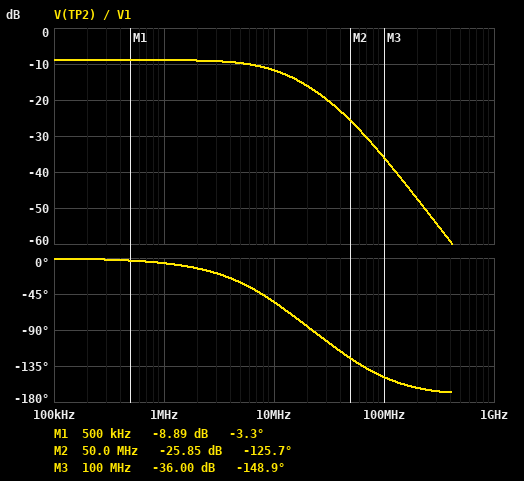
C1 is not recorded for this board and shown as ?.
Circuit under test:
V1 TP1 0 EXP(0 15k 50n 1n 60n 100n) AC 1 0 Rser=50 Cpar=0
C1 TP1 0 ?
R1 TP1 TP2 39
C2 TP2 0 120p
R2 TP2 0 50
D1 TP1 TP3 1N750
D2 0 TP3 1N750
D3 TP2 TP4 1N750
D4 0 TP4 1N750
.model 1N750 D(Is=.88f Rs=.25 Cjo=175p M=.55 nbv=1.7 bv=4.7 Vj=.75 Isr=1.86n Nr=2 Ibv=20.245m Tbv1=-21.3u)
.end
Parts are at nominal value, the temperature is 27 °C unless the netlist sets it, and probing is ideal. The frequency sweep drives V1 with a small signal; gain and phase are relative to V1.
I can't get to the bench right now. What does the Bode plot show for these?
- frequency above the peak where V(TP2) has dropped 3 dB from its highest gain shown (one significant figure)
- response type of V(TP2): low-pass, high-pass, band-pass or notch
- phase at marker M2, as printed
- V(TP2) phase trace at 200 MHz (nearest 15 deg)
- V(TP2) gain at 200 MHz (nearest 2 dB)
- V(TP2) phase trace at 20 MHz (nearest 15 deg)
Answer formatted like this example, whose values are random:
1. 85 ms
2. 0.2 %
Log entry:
1. 10 MHz
2. low-pass
3. -125.7 deg
4. -165 deg
5. -48 dB
6. -90 deg
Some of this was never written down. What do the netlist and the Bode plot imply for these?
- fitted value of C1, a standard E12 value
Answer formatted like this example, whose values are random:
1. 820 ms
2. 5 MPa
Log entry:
1. 270 pF
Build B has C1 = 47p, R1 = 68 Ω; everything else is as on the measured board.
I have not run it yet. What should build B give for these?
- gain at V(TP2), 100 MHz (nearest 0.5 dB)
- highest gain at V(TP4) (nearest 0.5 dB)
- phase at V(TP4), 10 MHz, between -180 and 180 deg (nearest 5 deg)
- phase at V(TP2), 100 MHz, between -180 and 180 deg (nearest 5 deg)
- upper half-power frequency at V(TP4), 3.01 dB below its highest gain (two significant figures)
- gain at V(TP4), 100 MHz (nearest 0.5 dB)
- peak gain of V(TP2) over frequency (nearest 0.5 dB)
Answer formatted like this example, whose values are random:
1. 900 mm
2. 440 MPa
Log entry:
1. -32.5 dB
2. -16.5 dB
3. -40 deg
4. -140 deg
5. 16 MHz
6. -38.5 dB
7. -10.5 dB
